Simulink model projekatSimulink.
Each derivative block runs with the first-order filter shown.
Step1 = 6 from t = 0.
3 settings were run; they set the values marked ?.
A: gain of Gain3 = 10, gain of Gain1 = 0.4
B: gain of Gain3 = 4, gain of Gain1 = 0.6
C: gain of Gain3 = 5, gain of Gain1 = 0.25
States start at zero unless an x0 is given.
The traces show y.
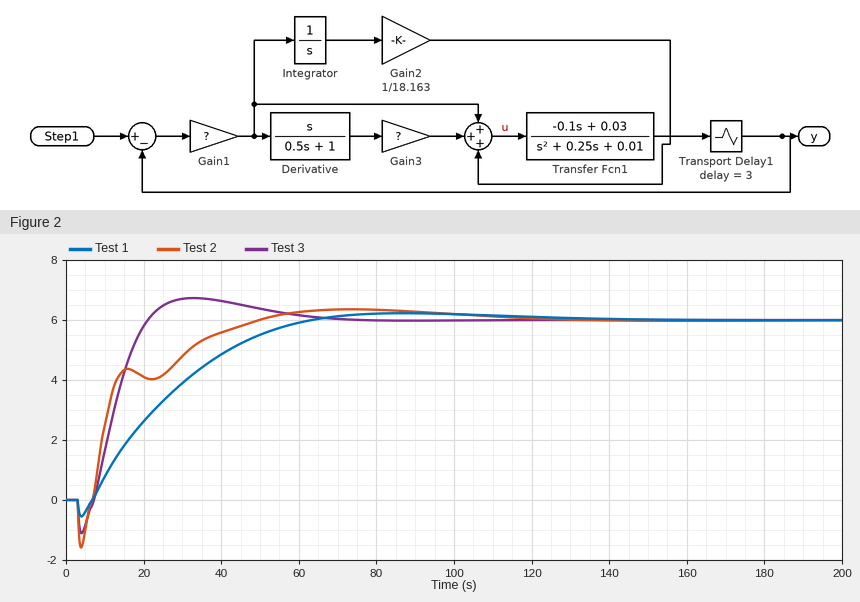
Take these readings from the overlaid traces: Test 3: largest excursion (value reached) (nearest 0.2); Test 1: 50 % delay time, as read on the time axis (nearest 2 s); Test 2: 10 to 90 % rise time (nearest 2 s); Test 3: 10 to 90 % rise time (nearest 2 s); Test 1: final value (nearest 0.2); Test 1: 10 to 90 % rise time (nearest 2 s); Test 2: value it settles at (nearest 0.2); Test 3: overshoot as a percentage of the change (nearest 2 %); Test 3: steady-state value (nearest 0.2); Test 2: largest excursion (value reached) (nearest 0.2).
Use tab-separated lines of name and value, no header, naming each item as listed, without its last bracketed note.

Test 3: largest excursion (value reached)	6.8
Test 1: 50 % delay time, as read on the time axis	22 s
Test 2: 10 to 90 % rise time	28 s
Test 3: 10 to 90 % rise time	10 s
Test 1: final value	6.0
Test 1: 10 to 90 % rise time	38 s
Test 2: value it settles at	6.0
Test 3: overshoot as a percentage of the change	12 %
Test 3: steady-state value	6.0
Test 2: largest excursion (value reached)	6.4
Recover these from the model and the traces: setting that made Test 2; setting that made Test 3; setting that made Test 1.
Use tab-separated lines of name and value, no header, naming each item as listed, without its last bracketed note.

setting that made Test 2	A
setting that made Test 3	B
setting that made Test 1	C
